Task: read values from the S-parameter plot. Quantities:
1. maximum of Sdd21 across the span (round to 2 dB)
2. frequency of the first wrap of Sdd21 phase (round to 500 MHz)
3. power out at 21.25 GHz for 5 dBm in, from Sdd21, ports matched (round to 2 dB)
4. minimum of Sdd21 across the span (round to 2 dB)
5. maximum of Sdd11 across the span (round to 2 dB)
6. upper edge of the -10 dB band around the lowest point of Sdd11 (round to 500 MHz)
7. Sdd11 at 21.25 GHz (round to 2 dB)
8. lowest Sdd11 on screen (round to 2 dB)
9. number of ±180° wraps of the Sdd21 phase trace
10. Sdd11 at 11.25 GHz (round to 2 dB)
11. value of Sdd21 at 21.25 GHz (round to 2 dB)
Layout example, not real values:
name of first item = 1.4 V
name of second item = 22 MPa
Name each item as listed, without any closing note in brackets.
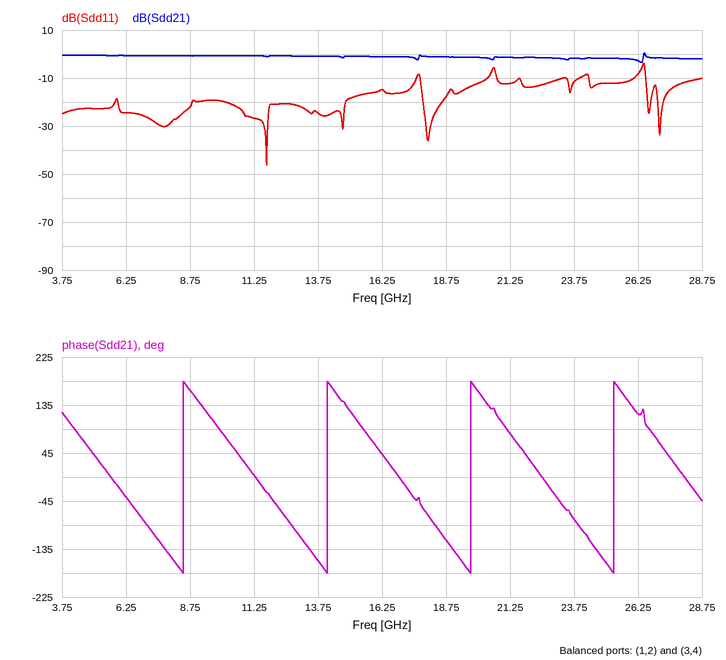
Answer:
maximum of Sdd21 across the span = 0 dB
frequency of the first wrap of Sdd21 phase = 8.5 GHz
power out at 21.25 GHz for 5 dBm in, from Sdd21, ports matched = 4 dBm
minimum of Sdd21 across the span = -4 dB
maximum of Sdd11 across the span = -4 dB
upper edge of the -10 dB band around the lowest point of Sdd11 = 17.5 GHz
Sdd11 at 21.25 GHz = -12 dB
lowest Sdd11 on screen = -46 dB
number of ±180° wraps of the Sdd21 phase trace = 4
Sdd11 at 11.25 GHz = -26 dB
value of Sdd21 at 21.25 GHz = -2 dB
